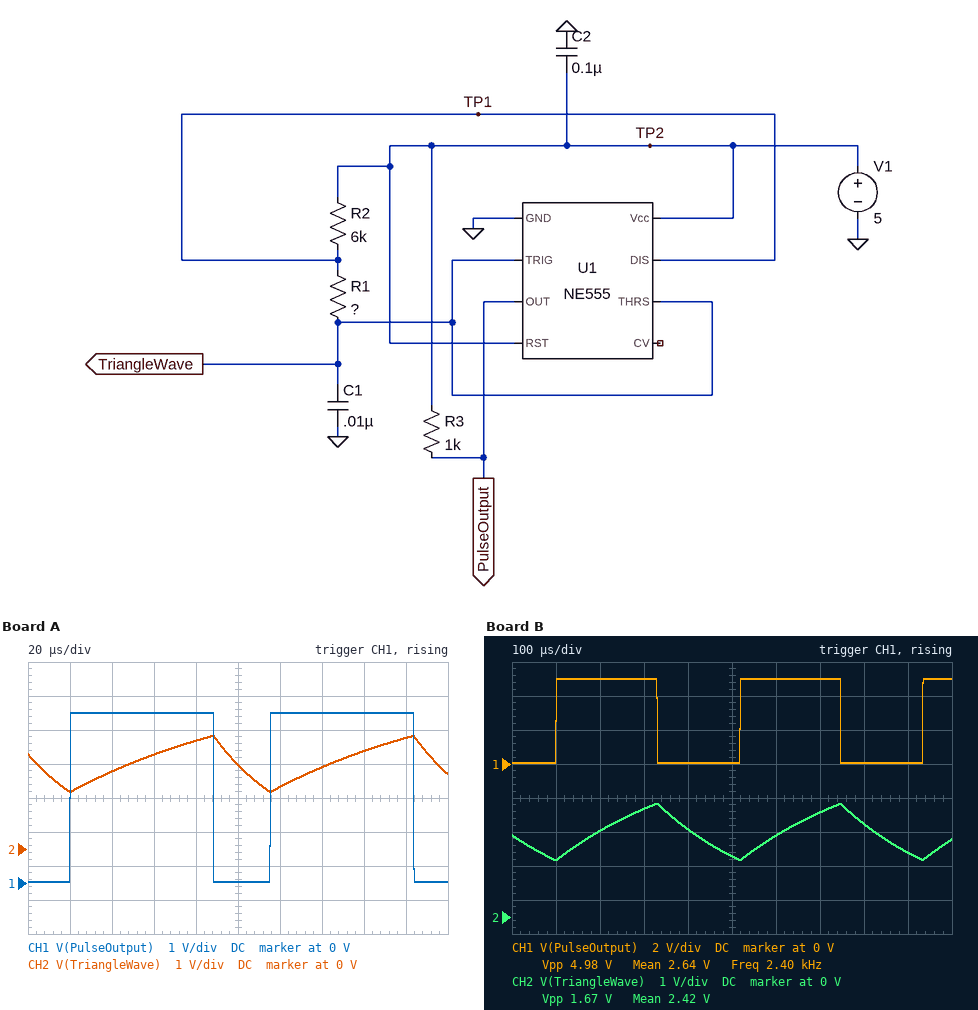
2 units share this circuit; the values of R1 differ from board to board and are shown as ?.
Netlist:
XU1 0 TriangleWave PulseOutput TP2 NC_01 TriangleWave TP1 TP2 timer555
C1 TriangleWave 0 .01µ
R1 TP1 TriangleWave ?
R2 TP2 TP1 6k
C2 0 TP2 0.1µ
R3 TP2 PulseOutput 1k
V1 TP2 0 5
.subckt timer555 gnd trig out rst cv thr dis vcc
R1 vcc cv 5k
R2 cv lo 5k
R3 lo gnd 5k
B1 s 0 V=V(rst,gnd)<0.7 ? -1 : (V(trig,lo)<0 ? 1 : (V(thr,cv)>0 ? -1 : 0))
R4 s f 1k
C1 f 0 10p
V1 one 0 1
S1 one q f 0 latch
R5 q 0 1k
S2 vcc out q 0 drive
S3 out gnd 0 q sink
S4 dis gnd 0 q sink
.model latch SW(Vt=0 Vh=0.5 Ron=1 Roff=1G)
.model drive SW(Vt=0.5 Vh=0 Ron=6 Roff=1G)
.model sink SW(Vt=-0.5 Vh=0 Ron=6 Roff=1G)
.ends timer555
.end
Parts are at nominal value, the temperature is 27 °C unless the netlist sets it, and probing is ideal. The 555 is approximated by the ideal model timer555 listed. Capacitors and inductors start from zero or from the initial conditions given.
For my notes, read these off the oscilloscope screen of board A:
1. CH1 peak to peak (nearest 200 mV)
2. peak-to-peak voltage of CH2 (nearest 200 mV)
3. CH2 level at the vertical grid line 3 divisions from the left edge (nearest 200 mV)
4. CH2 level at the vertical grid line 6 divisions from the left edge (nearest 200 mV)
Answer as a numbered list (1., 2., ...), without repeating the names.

1. 5.0 V
2. 1.6 V
3. 2.8 V
4. 1.8 V
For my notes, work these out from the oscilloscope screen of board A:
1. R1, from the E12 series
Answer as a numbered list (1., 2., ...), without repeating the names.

1. 3.9 kΩ
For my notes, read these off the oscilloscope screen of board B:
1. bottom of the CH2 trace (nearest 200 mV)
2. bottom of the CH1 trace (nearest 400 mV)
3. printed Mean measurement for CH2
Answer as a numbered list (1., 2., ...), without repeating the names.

1. 1.6 V
2. 0 V
3. 2.42 V
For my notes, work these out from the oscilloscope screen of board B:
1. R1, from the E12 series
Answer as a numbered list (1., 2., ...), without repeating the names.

1. 27 kΩ
